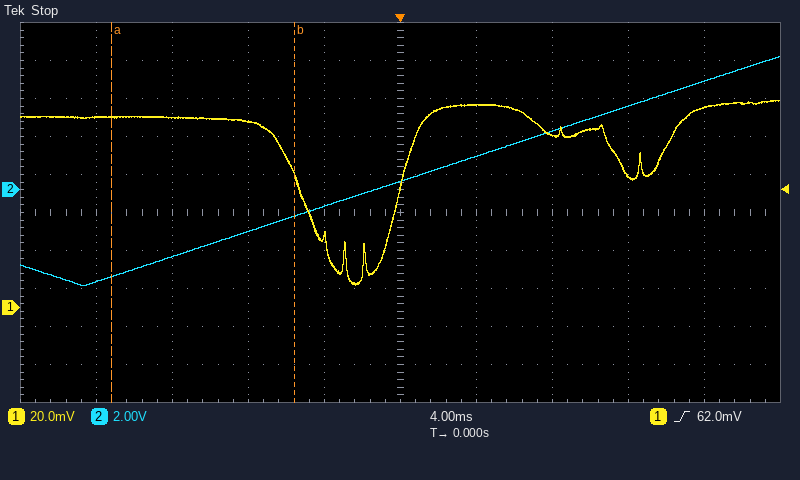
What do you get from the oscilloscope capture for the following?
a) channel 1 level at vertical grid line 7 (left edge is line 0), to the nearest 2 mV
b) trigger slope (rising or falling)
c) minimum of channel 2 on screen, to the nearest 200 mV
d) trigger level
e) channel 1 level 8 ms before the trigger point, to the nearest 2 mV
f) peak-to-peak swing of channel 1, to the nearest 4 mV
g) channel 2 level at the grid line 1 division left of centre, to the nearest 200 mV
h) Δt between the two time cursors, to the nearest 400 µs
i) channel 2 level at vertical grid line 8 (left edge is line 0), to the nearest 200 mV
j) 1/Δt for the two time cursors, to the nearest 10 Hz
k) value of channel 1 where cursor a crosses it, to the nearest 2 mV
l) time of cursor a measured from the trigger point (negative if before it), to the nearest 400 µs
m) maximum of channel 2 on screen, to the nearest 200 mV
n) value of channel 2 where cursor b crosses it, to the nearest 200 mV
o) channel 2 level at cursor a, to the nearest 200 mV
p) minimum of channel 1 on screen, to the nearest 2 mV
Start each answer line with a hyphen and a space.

- 90 mV
- rising
- -5.0 V
- 62.0 mV
- 98 mV
- 96 mV
- -800 mV
- 9.6 ms
- 4.4 V
- 100 Hz
- 100 mV
- -15.2 ms
- 7.0 V
- -1.4 V
- -4.6 V
- 12 mV
